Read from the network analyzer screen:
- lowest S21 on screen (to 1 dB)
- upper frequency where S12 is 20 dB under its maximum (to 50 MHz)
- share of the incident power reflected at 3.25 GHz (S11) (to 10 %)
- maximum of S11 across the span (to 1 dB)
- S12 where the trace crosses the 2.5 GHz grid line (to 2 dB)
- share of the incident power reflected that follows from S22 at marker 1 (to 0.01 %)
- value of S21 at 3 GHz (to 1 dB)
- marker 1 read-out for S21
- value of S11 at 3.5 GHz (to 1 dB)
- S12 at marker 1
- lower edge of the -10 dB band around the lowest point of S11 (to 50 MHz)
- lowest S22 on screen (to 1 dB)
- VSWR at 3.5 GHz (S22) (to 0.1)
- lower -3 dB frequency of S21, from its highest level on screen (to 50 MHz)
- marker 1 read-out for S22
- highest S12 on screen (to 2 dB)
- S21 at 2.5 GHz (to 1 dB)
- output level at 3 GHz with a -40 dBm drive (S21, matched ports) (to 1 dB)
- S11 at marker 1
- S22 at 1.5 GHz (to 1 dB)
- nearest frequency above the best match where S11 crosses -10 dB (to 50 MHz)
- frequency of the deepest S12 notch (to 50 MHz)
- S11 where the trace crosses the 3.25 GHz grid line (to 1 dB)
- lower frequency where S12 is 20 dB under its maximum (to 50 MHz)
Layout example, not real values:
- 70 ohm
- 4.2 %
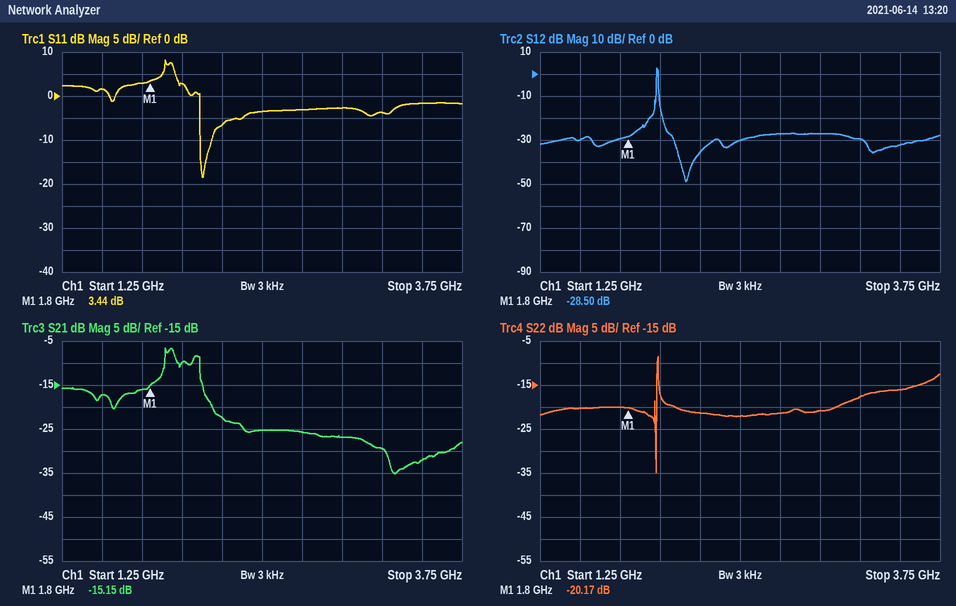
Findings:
- -35 dB
- 2.00 GHz
- 40 %
- 8 dB
- -30 dB
- 0.96 %
- -27 dB
- -15.15 dB
- -2 dB
- -28.50 dB
- 2.10 GHz
- -35 dB
- 1.4
- 1.90 GHz
- -20.17 dB
- 2 dB
- -25 dB
- -67 dBm
- 3.44 dB
- -20 dB
- 2.20 GHz
- 2.15 GHz
- -4 dB
- 1.95 GHz
